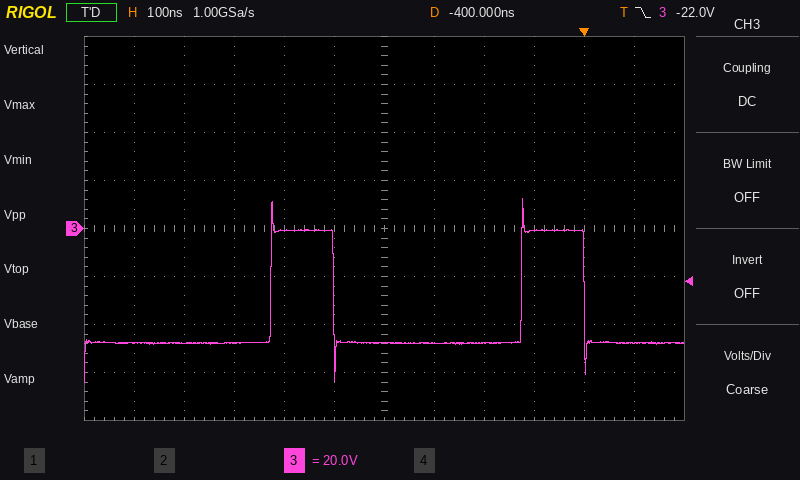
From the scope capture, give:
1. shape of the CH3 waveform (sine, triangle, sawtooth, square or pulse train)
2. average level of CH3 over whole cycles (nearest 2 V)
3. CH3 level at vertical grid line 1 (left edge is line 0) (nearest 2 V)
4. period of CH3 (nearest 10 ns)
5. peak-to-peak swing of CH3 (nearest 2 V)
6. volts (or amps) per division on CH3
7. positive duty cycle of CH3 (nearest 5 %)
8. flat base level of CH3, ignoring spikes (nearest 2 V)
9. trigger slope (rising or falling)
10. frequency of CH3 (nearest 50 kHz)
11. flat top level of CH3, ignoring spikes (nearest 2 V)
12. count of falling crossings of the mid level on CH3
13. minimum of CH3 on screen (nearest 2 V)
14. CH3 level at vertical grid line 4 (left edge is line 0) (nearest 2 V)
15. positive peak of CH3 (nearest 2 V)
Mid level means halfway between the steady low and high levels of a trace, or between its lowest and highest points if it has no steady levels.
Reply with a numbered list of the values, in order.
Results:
1. pulse train
2. -36 V
3. -48 V
4. 500 ns
5. 76 V
6. 20 V
7. 25 %
8. -48 V
9. falling
10. 2.00 MHz
11. 0 V
12. 2
13. -64 V
14. 0 V
15. 12 V
